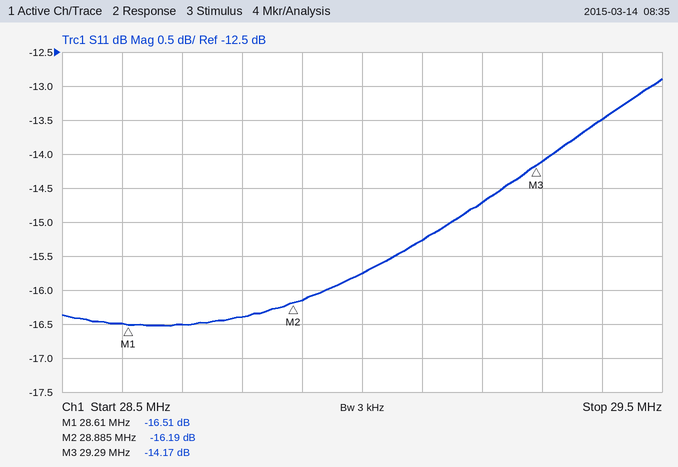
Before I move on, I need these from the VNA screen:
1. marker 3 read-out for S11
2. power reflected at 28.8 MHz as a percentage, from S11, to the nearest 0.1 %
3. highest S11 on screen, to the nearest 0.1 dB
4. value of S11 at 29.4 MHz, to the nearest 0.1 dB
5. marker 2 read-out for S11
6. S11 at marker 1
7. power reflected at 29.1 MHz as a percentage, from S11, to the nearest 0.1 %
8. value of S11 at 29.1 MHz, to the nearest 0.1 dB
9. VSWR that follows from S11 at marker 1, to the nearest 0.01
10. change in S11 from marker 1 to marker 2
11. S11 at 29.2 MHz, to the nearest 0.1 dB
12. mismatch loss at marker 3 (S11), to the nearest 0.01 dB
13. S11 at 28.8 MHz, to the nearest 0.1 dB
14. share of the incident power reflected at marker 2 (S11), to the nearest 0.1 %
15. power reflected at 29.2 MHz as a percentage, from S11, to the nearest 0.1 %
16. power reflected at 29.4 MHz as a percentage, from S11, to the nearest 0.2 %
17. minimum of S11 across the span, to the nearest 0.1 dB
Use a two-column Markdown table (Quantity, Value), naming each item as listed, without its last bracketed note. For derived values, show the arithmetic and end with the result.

| Quantity | Value |
|---|---|
| marker 3 read-out for S11 | -14.17 dB |
| power reflected at 28.8 MHz as a percentage, from S11, to the nearest 0.1 % | 10^(-16.4/10) ≈ 2.3 % |
| highest S11 on screen, to the nearest 0.1 dB | -12.9 dB |
| value of S11 at 29.4 MHz, to the nearest 0.1 dB | -13.5 dB |
| marker 2 read-out for S11 | -16.19 dB |
| S11 at marker 1 | -16.51 dB |
| power reflected at 29.1 MHz as a percentage, from S11, to the nearest 0.1 % | 10^(-15.3/10) ≈ 3.0 % |
| value of S11 at 29.1 MHz, to the nearest 0.1 dB | -15.3 dB |
| VSWR that follows from S11 at marker 1, to the nearest 0.01 | (1 + 0.1495)/(1 − 0.1495) ≈ 1.35 |
| change in S11 from marker 1 to marker 2 | -16.19 − (-16.51) = 0.32 dB |
| S11 at 29.2 MHz, to the nearest 0.1 dB | -14.7 dB |
| mismatch loss at marker 3 (S11), to the nearest 0.01 dB | −10 log10(1 − 10^(-14.17/10)) ≈ 0.17 dB |
| S11 at 28.8 MHz, to the nearest 0.1 dB | -16.4 dB |
| share of the incident power reflected at marker 2 (S11), to the nearest 0.1 % | 10^(-16.19/10) ≈ 2.4 % |
| power reflected at 29.2 MHz as a percentage, from S11, to the nearest 0.1 % | 10^(-14.7/10) ≈ 3.4 % |
| power reflected at 29.4 MHz as a percentage, from S11, to the nearest 0.2 % | 10^(-13.5/10) ≈ 4.47 %, so 4.4 % to the nearest 0.2 % |
| minimum of S11 across the span, to the nearest 0.1 dB | -16.5 dB |
